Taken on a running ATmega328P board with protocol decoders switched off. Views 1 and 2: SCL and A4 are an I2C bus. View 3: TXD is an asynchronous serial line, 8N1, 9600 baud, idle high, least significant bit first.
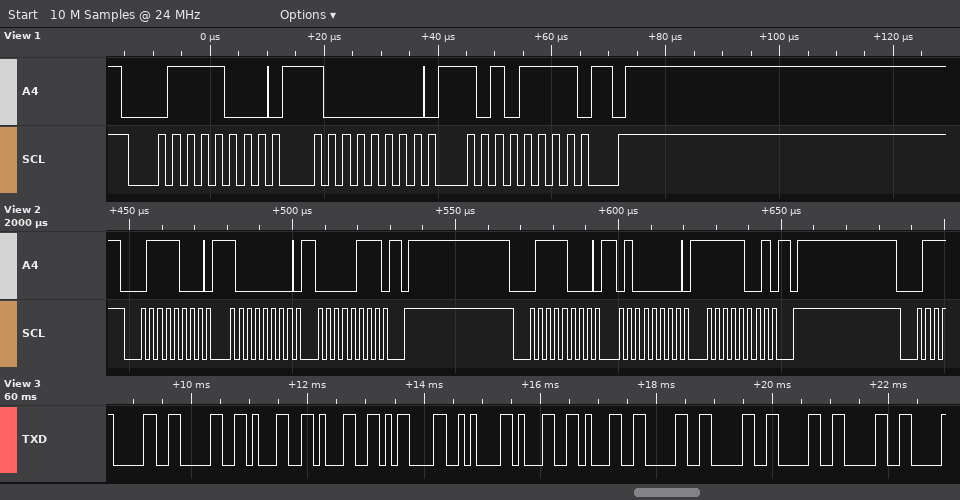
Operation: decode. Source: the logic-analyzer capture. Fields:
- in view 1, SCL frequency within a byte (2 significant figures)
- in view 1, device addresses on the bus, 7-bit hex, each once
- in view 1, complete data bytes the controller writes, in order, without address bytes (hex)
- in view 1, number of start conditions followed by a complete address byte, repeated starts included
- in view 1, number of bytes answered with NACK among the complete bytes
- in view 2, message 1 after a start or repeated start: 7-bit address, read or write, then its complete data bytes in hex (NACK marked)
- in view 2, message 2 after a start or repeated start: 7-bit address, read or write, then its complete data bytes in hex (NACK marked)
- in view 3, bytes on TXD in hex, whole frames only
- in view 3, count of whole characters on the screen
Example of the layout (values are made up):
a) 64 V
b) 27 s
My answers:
a) 400 kHz
b) 0x3C
c) 80 AF
d) 1
e) 0
f) 0x3C write: 80 07
g) 0x3C write: 40 F9
h) 30 30 31 31 0D 0A 31 31 30 30 30 30
i) 12
